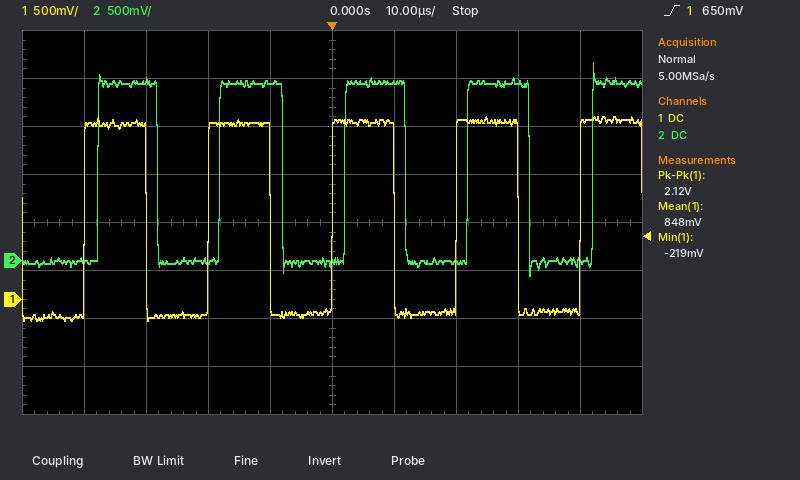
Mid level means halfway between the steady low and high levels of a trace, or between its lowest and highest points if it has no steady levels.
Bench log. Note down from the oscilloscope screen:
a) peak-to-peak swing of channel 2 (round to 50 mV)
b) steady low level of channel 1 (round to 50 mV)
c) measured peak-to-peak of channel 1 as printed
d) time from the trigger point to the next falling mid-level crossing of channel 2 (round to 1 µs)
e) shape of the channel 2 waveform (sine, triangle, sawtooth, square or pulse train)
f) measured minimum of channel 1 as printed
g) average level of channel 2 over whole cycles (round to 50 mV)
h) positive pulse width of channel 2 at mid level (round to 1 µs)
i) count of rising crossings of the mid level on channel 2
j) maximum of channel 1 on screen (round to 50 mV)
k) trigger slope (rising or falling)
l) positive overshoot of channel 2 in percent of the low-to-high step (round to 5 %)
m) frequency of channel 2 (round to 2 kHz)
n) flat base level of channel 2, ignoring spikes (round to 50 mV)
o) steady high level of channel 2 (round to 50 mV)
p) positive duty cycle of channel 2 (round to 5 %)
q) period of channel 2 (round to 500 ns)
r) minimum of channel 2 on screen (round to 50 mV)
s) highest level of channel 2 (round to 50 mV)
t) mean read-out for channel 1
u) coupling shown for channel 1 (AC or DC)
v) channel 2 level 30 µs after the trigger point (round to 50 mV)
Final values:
2.20 V
-150 mV
2.12 V
12 µs
square
-219 mV
900 mV
10 µs
5
1.90 V
rising
10 %
50 kHz
0 mV
1.85 V
50 %
20.0 µs
-150 mV
2.05 V
848 mV
DC
1.85 V
